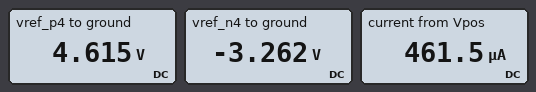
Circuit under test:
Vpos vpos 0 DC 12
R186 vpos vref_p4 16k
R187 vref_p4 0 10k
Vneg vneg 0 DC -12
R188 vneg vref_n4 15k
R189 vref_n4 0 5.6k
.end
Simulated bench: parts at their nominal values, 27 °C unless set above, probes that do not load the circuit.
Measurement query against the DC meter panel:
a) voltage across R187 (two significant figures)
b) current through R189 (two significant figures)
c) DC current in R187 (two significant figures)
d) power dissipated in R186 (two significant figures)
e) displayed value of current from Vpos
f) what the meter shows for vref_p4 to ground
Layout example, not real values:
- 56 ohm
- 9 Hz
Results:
- 4.6 V
- 580 µA
- 460 µA
- 3.4 mW
- 461.5 µA
- 4.615 V
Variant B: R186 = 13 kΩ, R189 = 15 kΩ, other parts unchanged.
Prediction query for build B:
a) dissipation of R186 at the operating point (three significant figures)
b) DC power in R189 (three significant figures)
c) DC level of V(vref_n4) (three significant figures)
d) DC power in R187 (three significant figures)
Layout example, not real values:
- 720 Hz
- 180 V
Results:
- 3.54 mW
- 2.40 mW
- -6.00 V
- 2.72 mW
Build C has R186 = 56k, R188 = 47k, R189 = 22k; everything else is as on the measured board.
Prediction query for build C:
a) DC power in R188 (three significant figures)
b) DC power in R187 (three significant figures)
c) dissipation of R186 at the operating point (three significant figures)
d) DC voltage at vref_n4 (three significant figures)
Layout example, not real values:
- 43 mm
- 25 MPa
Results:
- 1.42 mW
- 331 µW
- 1.85 mW
- -3.83 V
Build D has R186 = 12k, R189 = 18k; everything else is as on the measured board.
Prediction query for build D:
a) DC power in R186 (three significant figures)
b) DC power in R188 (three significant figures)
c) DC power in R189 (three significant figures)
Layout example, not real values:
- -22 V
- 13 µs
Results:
- 3.57 mW
- 1.98 mW
- 2.38 mW
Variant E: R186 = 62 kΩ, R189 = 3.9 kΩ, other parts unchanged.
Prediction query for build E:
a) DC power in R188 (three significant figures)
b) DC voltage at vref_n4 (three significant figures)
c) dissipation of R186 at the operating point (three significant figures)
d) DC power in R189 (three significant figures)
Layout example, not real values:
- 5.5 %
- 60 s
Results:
- 6.05 mW
- -2.48 V
- 1.72 mW
- 1.57 mW
